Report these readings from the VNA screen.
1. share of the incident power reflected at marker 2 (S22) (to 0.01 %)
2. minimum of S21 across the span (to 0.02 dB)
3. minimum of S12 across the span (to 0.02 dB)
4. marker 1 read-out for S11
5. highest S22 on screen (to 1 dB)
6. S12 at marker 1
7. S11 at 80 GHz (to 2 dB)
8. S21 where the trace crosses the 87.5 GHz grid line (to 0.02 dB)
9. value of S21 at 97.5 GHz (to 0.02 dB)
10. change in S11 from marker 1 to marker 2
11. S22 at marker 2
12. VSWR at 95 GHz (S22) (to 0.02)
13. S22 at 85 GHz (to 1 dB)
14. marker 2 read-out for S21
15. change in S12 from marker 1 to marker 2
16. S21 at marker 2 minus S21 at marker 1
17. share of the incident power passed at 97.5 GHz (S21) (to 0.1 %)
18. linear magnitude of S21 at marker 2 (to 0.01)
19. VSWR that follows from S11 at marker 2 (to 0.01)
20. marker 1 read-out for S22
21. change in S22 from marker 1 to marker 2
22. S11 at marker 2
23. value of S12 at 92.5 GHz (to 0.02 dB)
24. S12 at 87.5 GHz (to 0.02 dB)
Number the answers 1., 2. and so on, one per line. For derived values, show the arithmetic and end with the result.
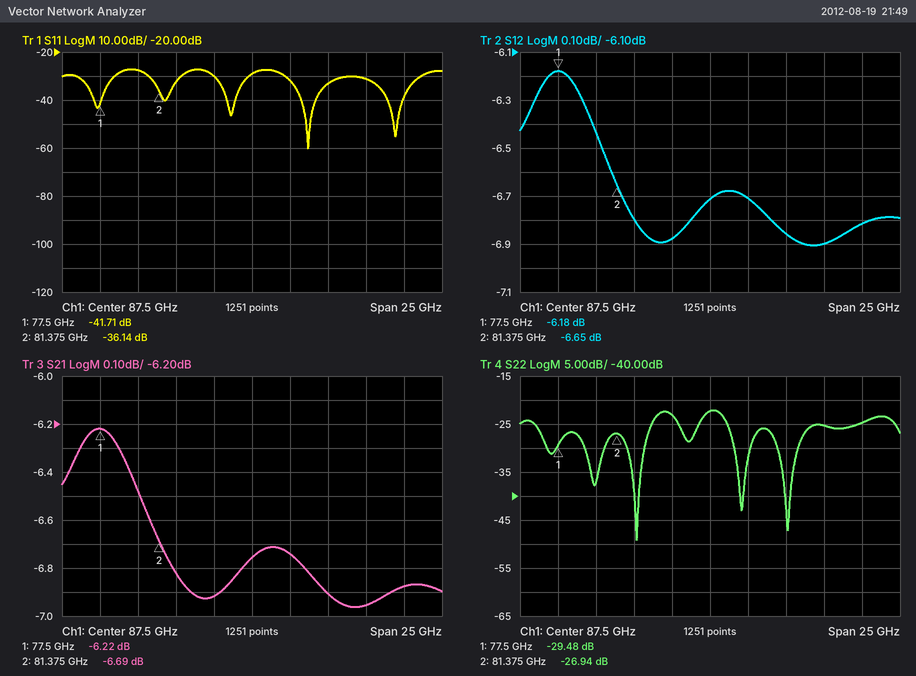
1. 10^(-26.94/10) ≈ 0.20 %
2. -6.96 dB
3. -6.90 dB
4. -41.71 dB
5. -22 dB
6. -6.18 dB
7. -28 dB
8. -6.76 dB
9. -6.88 dB
10. -36.14 − (-41.71) = 5.57 dB
11. -26.94 dB
12. |Γ| = 10^(-25/20) = 0.0562; VSWR = (1 + 0.0562)/(1 − 0.0562) ≈ 1.12
13. -23 dB
14. -6.69 dB
15. -6.65 − (-6.18) = -0.47 dB
16. -6.69 − (-6.22) = -0.47 dB
17. 10^(-6.88/10) ≈ 20.5 %
18. 10^(-6.69/20) ≈ 0.46
19. (1 + 0.0156)/(1 − 0.0156) ≈ 1.03
20. -29.48 dB
21. -26.94 − (-29.48) = 2.54 dB
22. -36.14 dB
23. -6.86 dB
24. -6.72 dB
